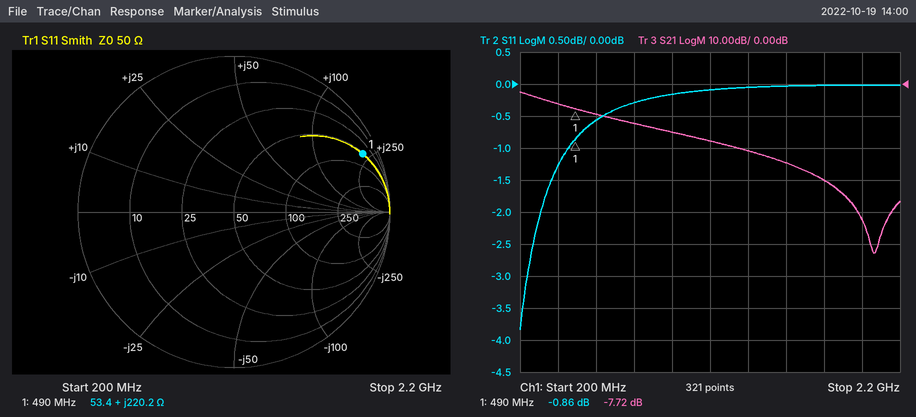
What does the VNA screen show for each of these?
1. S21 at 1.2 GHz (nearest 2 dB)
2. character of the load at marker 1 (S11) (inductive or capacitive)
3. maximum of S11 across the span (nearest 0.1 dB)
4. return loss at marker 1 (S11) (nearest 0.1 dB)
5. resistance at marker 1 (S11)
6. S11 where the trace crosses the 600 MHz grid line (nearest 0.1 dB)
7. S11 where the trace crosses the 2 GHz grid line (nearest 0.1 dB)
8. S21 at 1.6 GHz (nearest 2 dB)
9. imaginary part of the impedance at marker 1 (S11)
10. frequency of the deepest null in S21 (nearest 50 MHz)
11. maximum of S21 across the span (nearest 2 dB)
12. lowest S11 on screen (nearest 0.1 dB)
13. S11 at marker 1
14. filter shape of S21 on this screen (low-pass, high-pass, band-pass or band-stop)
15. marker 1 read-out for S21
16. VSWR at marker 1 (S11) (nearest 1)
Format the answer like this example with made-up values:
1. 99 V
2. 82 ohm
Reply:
1. -18 dB
2. inductive
3. 0.0 dB
4. 0.9 dB
5. 53.4 Ω
6. -0.6 dB
7. 0.0 dB
8. -24 dB
9. +220.2 Ω
10. 2.05 GHz
11. -2 dB
12. -3.8 dB
13. -0.86 dB
14. low-pass
15. -7.72 dB
16. 20
